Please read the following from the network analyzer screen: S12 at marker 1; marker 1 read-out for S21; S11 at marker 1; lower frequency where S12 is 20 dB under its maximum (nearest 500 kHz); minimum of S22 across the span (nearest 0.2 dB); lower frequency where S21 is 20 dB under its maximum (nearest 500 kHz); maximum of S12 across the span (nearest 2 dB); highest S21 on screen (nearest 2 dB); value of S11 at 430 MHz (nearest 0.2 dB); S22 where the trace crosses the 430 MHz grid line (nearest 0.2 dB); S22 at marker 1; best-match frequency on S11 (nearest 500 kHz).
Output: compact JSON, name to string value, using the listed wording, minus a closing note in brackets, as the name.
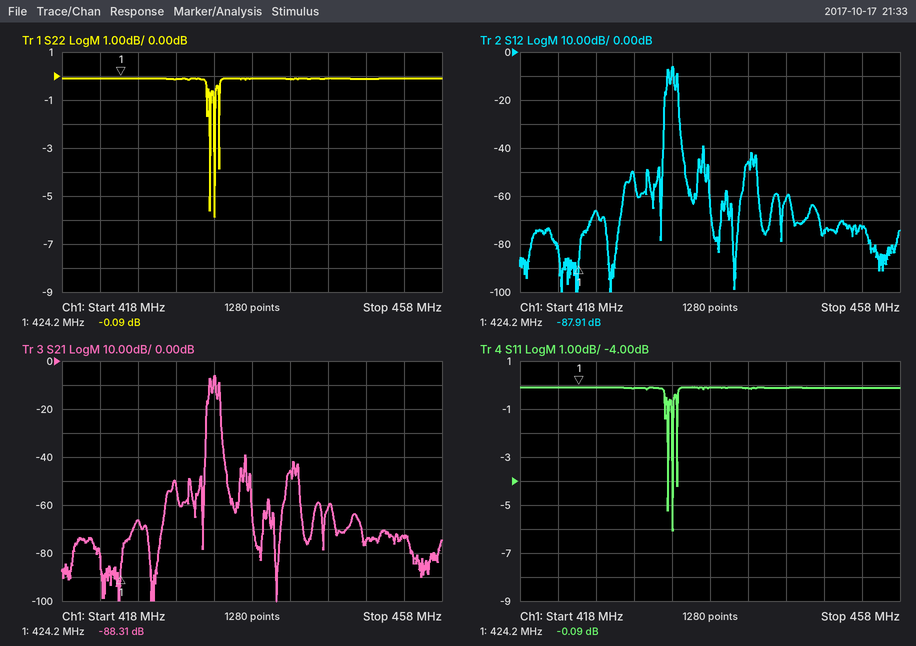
{"S12 at marker 1": "-87.91 dB", "marker 1 read-out for S21": "-88.31 dB", "S11 at marker 1": "-0.09 dB", "lower frequency where S12 is 20 dB under its maximum": "433.0 MHz", "minimum of S22 across the span": "-5.8 dB", "lower frequency where S21 is 20 dB under its maximum": "433.0 MHz", "maximum of S12 across the span": "-6 dB", "highest S21 on screen": "-6 dB", "value of S11 at 430 MHz": "-0.2 dB", "S22 where the trace crosses the 430 MHz grid line": "-0.2 dB", "S22 at marker 1": "-0.09 dB", "best-match frequency on S11": "434.0 MHz"}
